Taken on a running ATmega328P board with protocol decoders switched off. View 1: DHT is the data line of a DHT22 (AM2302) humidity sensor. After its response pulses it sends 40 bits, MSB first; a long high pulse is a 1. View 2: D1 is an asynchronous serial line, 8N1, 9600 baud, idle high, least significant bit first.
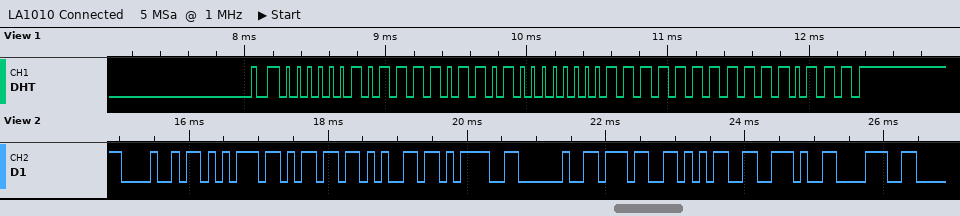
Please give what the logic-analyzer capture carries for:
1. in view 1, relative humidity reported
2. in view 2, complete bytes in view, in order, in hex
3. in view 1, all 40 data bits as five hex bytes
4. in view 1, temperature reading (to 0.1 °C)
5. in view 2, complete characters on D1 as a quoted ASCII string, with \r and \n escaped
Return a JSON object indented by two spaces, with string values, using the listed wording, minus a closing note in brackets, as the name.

{
  "in view 1, relative humidity reported": "75.8 %",
  "in view 2, complete bytes in view, in order, in hex": "48 75 6D 65 3D 20 37 35 2E 38",
  "in view 1, all 40 data bits as five hex bytes": "02 F6 80 7F F7",
  "in view 1, temperature reading": "-12.7 °C",
  "in view 2, complete characters on D1 as a quoted ASCII string, with \\r and \\n escaped": "\"Hume= 75.8\""
}
